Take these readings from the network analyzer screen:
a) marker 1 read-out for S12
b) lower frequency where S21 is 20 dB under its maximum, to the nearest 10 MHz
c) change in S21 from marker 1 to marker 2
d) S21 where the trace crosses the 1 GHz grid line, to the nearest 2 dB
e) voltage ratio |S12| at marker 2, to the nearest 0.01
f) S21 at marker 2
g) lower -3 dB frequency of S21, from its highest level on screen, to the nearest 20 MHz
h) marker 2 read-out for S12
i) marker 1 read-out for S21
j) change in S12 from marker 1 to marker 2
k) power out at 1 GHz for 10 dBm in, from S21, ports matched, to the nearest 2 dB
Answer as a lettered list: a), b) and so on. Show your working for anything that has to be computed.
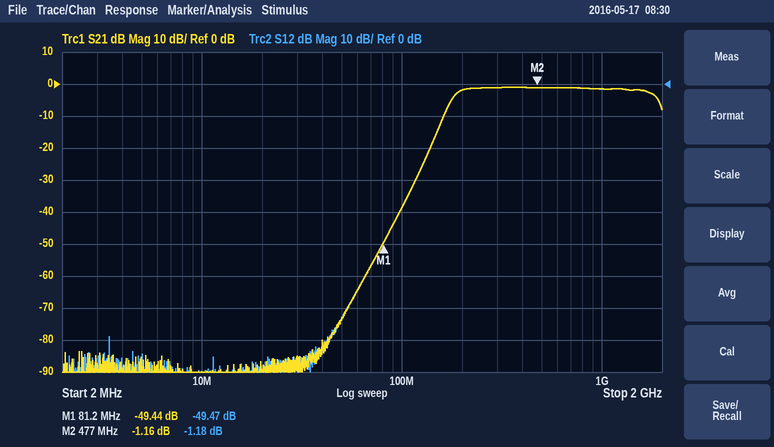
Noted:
a) -49.47 dB
b) 140 MHz
c) -1.16 − (-49.44) = 48.28 dB
d) -2 dB
e) 10^(-1.18/20) ≈ 0.87
f) -1.16 dB
g) 180 MHz
h) -1.18 dB
i) -49.44 dB
j) -1.18 − (-49.47) = 48.29 dB
k) 10 dBm + (-2 dB) = 8 dBm
